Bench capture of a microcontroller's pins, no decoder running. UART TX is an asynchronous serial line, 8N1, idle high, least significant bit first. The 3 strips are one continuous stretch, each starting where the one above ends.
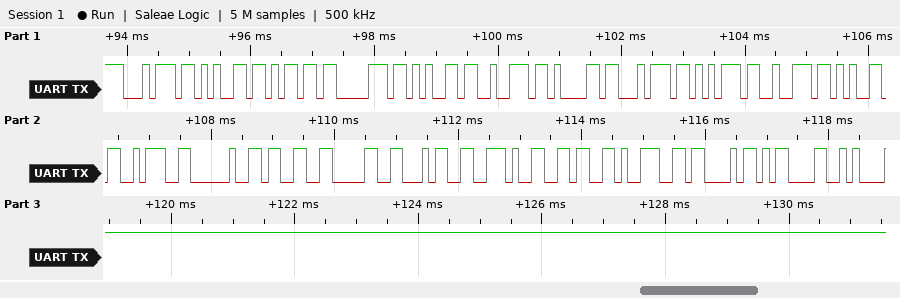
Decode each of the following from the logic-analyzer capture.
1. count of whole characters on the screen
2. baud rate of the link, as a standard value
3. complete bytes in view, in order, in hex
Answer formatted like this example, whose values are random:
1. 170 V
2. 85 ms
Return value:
1. 22
2. 9600 baud
3. 74 65 6D 70 65 72 61 74 75 72 65 3A 20 33 30 34 2E 36 39 43 0D 0A
